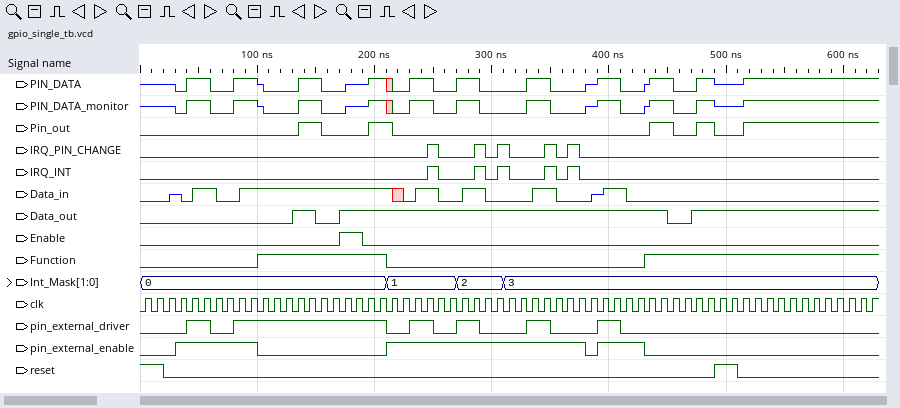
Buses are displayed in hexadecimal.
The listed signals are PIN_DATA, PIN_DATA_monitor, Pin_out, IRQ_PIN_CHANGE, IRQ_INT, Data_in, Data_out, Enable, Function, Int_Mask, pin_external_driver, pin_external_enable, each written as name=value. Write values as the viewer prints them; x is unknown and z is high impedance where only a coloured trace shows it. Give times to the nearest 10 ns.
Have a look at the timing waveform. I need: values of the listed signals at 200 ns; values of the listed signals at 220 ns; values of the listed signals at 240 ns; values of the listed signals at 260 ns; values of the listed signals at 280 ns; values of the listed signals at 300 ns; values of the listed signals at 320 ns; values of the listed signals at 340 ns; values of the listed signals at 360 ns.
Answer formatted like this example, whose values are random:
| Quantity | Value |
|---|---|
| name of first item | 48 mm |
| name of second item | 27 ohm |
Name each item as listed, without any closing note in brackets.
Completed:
| Quantity | Value |
|---|---|
| values of the listed signals at 200 ns | PIN_DATA=1, PIN_DATA_monitor=1, Pin_out=1, IRQ_PIN_CHANGE=0, IRQ_INT=0, Data_in=1, Data_out=1, Enable=0, Function=1, Int_Mask=0, pin_external_driver=1, pin_external_enable=0 |
| values of the listed signals at 220 ns | PIN_DATA=0, PIN_DATA_monitor=0, Pin_out=0, IRQ_PIN_CHANGE=0, IRQ_INT=0, Data_in=x, Data_out=1, Enable=0, Function=0, Int_Mask=1, pin_external_driver=0, pin_external_enable=1 |
| values of the listed signals at 240 ns | PIN_DATA=1, PIN_DATA_monitor=1, Pin_out=0, IRQ_PIN_CHANGE=0, IRQ_INT=0, Data_in=1, Data_out=1, Enable=0, Function=0, Int_Mask=1, pin_external_driver=1, pin_external_enable=1 |
| values of the listed signals at 260 ns | PIN_DATA=0, PIN_DATA_monitor=0, Pin_out=0, IRQ_PIN_CHANGE=0, IRQ_INT=0, Data_in=0, Data_out=1, Enable=0, Function=0, Int_Mask=1, pin_external_driver=0, pin_external_enable=1 |
| values of the listed signals at 280 ns | PIN_DATA=1, PIN_DATA_monitor=1, Pin_out=0, IRQ_PIN_CHANGE=0, IRQ_INT=0, Data_in=1, Data_out=1, Enable=0, Function=0, Int_Mask=2, pin_external_driver=1, pin_external_enable=1 |
| values of the listed signals at 300 ns | PIN_DATA=0, PIN_DATA_monitor=0, Pin_out=0, IRQ_PIN_CHANGE=0, IRQ_INT=0, Data_in=0, Data_out=1, Enable=0, Function=0, Int_Mask=2, pin_external_driver=0, pin_external_enable=1 |
| values of the listed signals at 320 ns | PIN_DATA=0, PIN_DATA_monitor=0, Pin_out=0, IRQ_PIN_CHANGE=0, IRQ_INT=0, Data_in=0, Data_out=1, Enable=0, Function=0, Int_Mask=3, pin_external_driver=0, pin_external_enable=1 |
| values of the listed signals at 340 ns | PIN_DATA=1, PIN_DATA_monitor=1, Pin_out=0, IRQ_PIN_CHANGE=0, IRQ_INT=0, Data_in=1, Data_out=1, Enable=0, Function=0, Int_Mask=3, pin_external_driver=1, pin_external_enable=1 |
| values of the listed signals at 360 ns | PIN_DATA=0, PIN_DATA_monitor=0, Pin_out=0, IRQ_PIN_CHANGE=0, IRQ_INT=0, Data_in=0, Data_out=1, Enable=0, Function=0, Int_Mask=3, pin_external_driver=0, pin_external_enable=1 |
